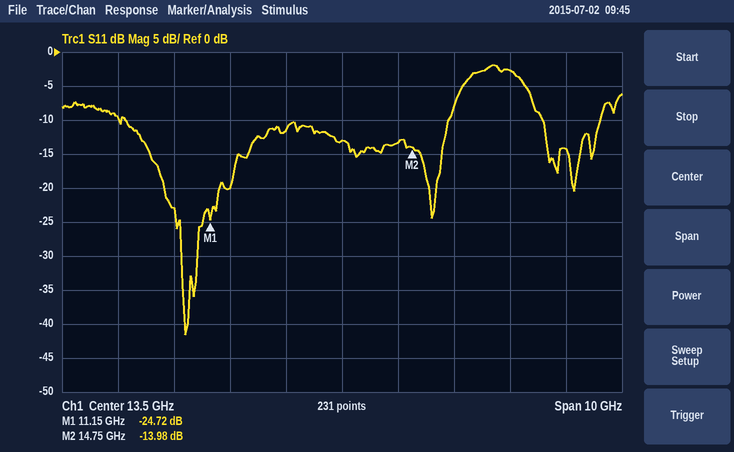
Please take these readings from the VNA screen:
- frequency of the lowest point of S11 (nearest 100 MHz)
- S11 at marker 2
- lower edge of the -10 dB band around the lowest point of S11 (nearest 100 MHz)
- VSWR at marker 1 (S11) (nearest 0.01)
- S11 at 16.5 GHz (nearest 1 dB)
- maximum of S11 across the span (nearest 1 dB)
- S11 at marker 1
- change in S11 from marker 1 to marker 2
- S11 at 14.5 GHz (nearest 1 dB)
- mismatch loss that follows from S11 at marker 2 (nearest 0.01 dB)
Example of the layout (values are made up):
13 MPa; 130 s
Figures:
10.7 GHz; -13.98 dB; 9.6 GHz; 1.12; -3 dB; -2 dB; -24.72 dB; 10.74 dB; -13 dB; 0.18 dB
